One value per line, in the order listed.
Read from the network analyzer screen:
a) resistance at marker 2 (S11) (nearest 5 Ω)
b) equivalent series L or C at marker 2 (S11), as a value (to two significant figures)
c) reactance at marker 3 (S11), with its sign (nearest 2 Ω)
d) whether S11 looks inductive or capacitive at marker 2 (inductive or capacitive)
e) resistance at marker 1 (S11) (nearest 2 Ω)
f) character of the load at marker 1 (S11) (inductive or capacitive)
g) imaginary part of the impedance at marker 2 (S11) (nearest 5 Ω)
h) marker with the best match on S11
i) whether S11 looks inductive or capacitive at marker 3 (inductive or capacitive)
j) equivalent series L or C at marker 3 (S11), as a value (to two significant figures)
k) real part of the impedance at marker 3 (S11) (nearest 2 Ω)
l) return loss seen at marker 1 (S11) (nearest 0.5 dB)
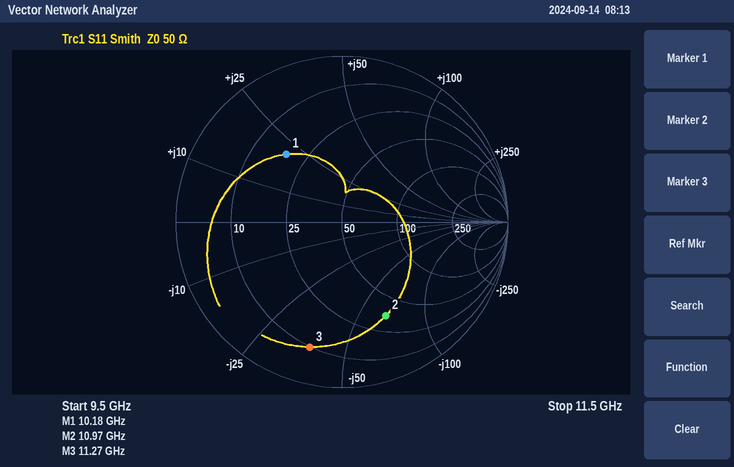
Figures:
35 Ω
220 fF
-38 Ω
capacitive
18 Ω
inductive
-65 Ω
marker 1
capacitive
370 fF
10 Ω
5.5 dB
